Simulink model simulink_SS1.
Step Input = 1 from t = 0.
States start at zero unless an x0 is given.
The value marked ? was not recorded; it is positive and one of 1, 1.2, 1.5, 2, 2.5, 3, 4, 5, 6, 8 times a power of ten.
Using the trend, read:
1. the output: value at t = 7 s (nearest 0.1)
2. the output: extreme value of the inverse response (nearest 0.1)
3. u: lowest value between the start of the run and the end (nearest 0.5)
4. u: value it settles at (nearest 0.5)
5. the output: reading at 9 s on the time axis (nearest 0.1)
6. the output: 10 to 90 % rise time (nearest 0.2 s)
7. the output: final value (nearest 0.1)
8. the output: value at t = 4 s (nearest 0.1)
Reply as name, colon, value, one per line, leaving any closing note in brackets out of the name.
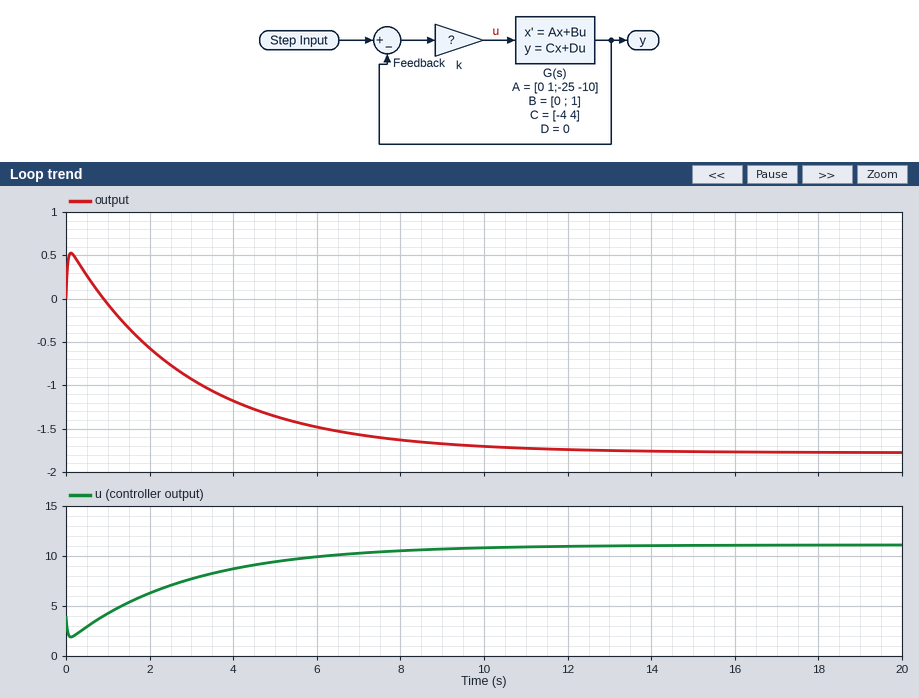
the output: value at t = 7 s: -1.6
the output: extreme value of the inverse response: 0.5
u: lowest value between the start of the run and the end: 2.0
u: value it settles at: 11.0
the output: reading at 9 s on the time axis: -1.7
the output: 10 to 90 % rise time: 6.2 s
the output: final value: -1.8
the output: value at t = 4 s: -1.2
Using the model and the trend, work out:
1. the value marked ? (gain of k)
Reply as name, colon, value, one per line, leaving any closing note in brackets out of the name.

the value marked ?: 4
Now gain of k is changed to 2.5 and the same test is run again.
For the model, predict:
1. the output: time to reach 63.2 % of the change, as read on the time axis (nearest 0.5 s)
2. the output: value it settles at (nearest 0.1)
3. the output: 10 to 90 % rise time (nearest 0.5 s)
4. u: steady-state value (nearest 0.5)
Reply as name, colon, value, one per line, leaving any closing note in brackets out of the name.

the output: time to reach 63.2 % of the change, as read on the time axis: 2.0 s
the output: value it settles at: -0.7
the output: 10 to 90 % rise time: 3.0 s
u: steady-state value: 4.0
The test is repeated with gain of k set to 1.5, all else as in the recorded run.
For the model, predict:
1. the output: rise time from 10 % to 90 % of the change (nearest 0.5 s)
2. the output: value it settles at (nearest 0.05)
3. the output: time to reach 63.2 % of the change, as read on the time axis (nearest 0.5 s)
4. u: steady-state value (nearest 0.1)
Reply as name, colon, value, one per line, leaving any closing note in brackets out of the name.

the output: rise time from 10 % to 90 % of the change: 1.5 s
the output: value it settles at: -0.30
the output: time to reach 63.2 % of the change, as read on the time axis: 1.5 s
u: steady-state value: 2.0
